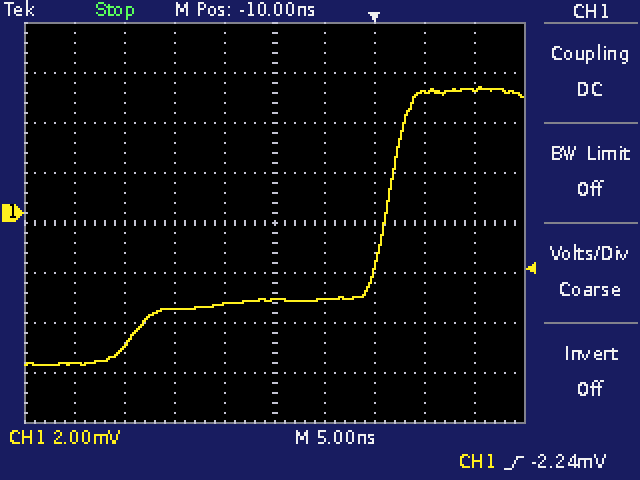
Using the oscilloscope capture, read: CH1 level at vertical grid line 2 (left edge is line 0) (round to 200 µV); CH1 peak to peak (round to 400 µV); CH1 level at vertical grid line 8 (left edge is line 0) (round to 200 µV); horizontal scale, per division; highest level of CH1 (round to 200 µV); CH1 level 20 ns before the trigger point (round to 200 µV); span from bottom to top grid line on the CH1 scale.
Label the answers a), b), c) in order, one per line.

a) -5.4 mV
b) 11.2 mV
c) 4.8 mV
d) 5 ns
e) 5.0 mV
f) -3.8 mV
g) 16 mV
